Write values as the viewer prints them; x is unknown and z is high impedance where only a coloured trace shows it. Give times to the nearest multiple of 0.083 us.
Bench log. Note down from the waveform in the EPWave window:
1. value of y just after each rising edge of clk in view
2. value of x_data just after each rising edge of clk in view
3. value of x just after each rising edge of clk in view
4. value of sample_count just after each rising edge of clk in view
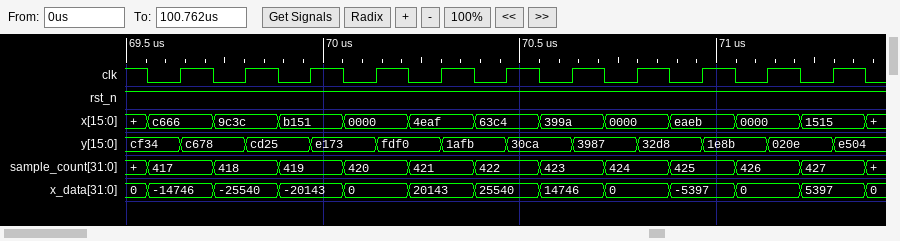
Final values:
c678, cd25, e173, fdf0, 1afb, 30ca, 3987, 32d8, 1e8b, 020e, e504
-14746, -25540, -20143, 0, 20143, 25540, 14746, 0, -5397, 0, 5397
c666, 9c3c, b151, 0000, 4eaf, 63c4, 399a, 0000, eaeb, 0000, 1515
417, 418, 419, 420, 421, 422, 423, 424, 425, 426, 427
